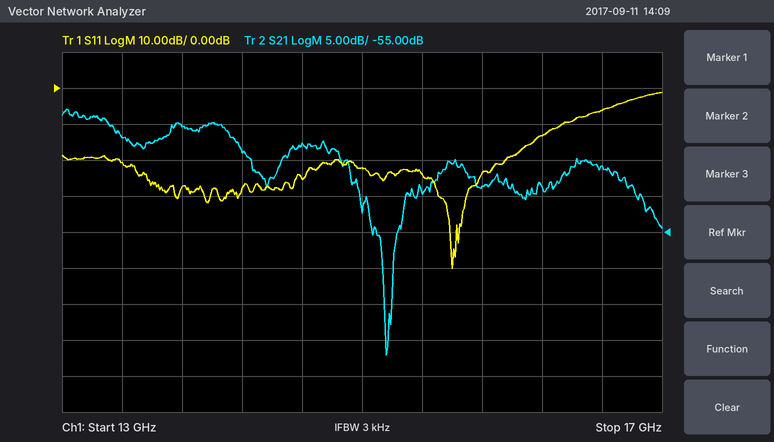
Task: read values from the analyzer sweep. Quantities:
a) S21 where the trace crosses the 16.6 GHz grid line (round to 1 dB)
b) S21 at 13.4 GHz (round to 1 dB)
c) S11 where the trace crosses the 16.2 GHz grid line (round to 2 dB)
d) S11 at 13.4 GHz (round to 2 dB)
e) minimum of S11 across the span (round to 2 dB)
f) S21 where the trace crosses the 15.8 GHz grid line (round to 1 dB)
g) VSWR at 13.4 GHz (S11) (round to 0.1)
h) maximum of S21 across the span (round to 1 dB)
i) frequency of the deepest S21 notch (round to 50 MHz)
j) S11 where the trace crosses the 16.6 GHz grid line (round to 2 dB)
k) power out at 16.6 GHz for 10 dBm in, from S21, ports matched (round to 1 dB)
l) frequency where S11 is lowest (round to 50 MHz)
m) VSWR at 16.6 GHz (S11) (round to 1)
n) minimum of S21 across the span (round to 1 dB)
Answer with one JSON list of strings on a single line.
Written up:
["-46 dB", "-42 dB", "-14 dB", "-20 dB", "-50 dB", "-49 dB", "1.2", "-38 dB", "15.15 GHz", "-6 dB", "-36 dBm", "15.60 GHz", "3", "-72 dB"]
